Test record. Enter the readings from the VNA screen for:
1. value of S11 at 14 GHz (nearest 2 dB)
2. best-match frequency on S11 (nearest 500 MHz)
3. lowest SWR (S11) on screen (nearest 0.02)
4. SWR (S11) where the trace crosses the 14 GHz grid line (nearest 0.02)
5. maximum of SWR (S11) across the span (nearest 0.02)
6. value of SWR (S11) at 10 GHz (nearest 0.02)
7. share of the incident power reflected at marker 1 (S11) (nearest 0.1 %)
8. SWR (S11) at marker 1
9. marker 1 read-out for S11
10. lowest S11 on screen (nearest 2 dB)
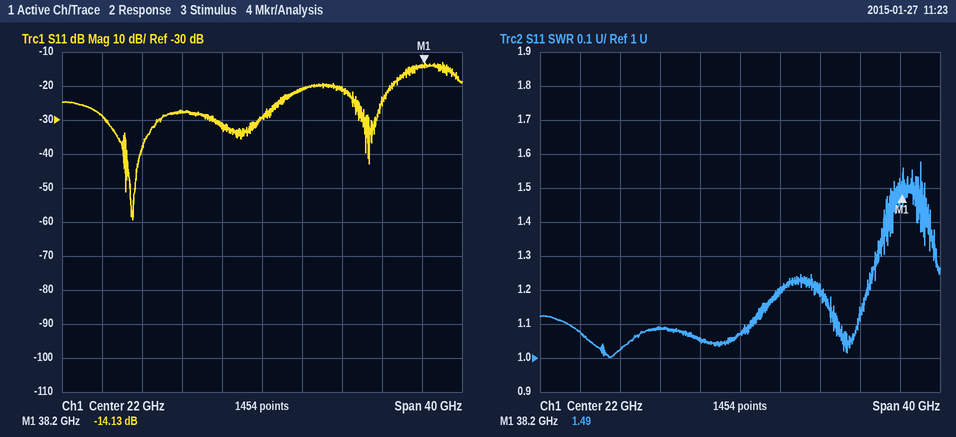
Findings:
-28 dB
9.0 GHz
1.00
1.08
1.58
1.02
3.9 %
1.49
-14.13 dB
-60 dB
